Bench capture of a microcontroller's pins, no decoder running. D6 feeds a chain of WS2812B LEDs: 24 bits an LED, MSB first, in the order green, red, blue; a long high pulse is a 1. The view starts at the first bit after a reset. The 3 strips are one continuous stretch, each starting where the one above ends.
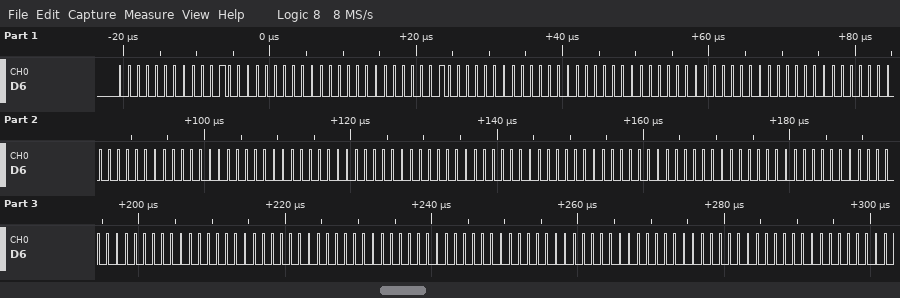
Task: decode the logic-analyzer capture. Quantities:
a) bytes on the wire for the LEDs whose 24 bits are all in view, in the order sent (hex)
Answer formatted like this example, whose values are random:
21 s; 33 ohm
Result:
00 10 00 00 10 00 00 00 00 00 00 00 00 00 00 00 00 00 00 00 00 00 00 00 00 00 00 00 00 00
